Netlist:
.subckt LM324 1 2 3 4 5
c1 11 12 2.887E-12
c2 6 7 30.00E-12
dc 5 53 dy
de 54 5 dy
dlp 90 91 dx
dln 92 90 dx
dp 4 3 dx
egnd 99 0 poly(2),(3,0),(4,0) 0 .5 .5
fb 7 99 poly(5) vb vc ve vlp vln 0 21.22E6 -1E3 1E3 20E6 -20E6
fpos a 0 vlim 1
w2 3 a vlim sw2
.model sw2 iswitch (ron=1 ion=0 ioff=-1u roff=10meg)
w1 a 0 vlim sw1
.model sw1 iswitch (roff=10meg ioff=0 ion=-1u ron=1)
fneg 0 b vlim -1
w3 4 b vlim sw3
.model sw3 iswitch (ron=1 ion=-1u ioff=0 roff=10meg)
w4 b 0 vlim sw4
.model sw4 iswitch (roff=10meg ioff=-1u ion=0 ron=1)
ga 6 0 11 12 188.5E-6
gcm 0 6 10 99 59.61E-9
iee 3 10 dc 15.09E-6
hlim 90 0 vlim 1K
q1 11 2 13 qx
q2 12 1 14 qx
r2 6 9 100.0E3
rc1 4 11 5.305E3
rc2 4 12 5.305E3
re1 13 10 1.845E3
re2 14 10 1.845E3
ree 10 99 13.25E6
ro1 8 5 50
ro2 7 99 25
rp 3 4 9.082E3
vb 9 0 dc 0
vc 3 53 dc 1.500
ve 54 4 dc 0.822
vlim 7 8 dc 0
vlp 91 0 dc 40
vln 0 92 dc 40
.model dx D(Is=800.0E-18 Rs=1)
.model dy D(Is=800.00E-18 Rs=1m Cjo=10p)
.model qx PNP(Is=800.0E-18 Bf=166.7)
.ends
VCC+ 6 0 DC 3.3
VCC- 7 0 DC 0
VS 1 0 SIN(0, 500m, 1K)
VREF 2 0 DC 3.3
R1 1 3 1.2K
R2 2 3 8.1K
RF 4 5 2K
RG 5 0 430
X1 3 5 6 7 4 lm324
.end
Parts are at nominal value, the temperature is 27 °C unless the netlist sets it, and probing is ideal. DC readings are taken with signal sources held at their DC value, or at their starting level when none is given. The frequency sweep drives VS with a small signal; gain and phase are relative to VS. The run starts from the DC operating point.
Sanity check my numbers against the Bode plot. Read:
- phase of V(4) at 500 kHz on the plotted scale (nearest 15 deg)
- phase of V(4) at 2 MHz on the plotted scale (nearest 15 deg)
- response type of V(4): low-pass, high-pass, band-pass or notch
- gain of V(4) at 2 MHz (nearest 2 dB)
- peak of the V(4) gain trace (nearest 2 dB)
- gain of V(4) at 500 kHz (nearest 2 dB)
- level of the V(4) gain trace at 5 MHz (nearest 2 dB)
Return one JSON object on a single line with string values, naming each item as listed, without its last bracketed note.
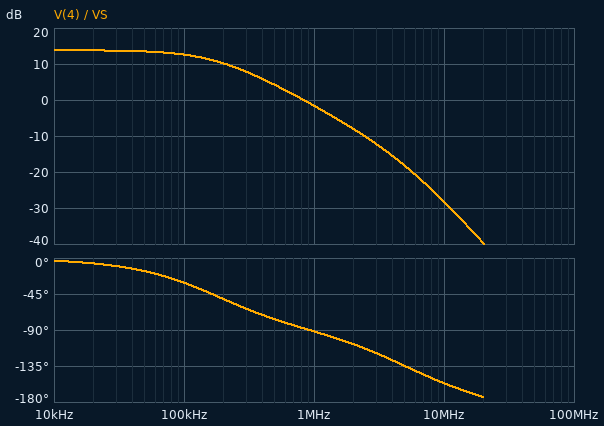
{"phase of V(4) at 500 kHz on the plotted scale": "-75 deg", "phase of V(4) at 2 MHz on the plotted scale": "-105 deg", "response type of V(4): low-pass, high-pass, band-pass or notch": "low-pass", "gain of V(4) at 2 MHz": "-8 dB", "peak of the V(4) gain trace": "14 dB", "gain of V(4) at 500 kHz": "4 dB", "level of the V(4) gain trace at 5 MHz": "-18 dB"}
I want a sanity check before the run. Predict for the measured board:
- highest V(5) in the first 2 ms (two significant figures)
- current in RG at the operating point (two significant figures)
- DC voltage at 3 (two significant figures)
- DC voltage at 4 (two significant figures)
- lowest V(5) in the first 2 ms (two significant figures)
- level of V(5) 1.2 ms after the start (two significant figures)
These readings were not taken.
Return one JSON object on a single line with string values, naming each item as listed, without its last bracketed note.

{"highest V(5) in the first 2 ms": "460 mV", "current in RG at the operating point": "990 µA", "DC voltage at 3": "430 mV", "DC voltage at 4": "2.4 V", "lowest V(5) in the first 2 ms": "1.8 mV", "level of V(5) 1.2 ms after the start": "460 mV"}
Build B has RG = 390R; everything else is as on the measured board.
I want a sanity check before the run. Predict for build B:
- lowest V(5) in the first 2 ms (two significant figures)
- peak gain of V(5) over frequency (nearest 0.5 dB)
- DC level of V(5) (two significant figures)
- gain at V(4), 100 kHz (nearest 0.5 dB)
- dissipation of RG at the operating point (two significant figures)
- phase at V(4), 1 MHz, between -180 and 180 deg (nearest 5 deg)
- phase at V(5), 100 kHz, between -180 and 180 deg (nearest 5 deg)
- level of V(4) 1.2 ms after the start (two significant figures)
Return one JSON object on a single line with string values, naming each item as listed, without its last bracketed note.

{"lowest V(5) in the first 2 ms": "1.7 mV", "peak gain of V(5) over frequency": "-6.5 dB", "DC level of V(5)": "420 mV", "gain at V(4), 100 kHz": "-11.0 dB", "dissipation of RG at the operating point": "460 µW", "phase at V(4), 1 MHz, between -180 and 180 deg": "-100 deg", "phase at V(5), 100 kHz, between -180 and 180 deg": "-85 deg", "level of V(4) 1.2 ms after the start": "2.6 V"}
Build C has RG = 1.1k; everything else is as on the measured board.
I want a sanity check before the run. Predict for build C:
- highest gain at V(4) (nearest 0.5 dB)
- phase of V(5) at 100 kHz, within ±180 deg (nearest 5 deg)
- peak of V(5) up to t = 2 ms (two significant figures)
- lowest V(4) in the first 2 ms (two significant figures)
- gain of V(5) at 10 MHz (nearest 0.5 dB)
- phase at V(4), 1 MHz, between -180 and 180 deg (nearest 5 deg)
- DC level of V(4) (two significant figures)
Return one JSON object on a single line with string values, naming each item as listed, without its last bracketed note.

{"highest gain at V(4)": "8.0 dB", "phase of V(5) at 100 kHz, within ±180 deg": "-15 deg", "peak of V(5) up to t = 2 ms": "860 mV", "lowest V(4) in the first 2 ms": "6.7 mV", "gain of V(5) at 10 MHz": "-37.0 dB", "phase at V(4), 1 MHz, between -180 and 180 deg": "-80 deg", "DC level of V(4)": "1.2 V"}
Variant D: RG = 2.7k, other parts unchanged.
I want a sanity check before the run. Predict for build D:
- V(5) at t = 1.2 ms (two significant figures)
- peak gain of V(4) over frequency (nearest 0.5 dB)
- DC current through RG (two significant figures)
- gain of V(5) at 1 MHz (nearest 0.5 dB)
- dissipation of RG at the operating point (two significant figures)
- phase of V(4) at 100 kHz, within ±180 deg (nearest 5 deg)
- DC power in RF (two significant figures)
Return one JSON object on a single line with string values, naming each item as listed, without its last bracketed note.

{"V(5) at t = 1.2 ms": "840 mV", "peak gain of V(4) over frequency": "3.5 dB", "DC current through RG": "160 µA", "gain of V(5) at 1 MHz": "-6.5 dB", "dissipation of RG at the operating point": "67 µW", "phase of V(4) at 100 kHz, within ±180 deg": "-10 deg", "DC power in RF": "50 µW"}
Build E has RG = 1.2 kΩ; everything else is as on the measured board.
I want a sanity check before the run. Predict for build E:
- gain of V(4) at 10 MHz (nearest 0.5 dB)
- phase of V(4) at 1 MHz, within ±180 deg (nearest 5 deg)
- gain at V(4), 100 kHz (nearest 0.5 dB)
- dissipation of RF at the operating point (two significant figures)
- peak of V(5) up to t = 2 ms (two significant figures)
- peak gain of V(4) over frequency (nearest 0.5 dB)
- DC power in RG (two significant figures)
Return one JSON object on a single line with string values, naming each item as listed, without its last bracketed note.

{"gain of V(4) at 10 MHz": "-28.0 dB", "phase of V(4) at 1 MHz, within ±180 deg": "-80 deg", "gain at V(4), 100 kHz": "7.0 dB", "dissipation of RF at the operating point": "250 µW", "peak of V(5) up to t = 2 ms": "860 mV", "peak gain of V(4) over frequency": "7.5 dB", "DC power in RG": "150 µW"}
